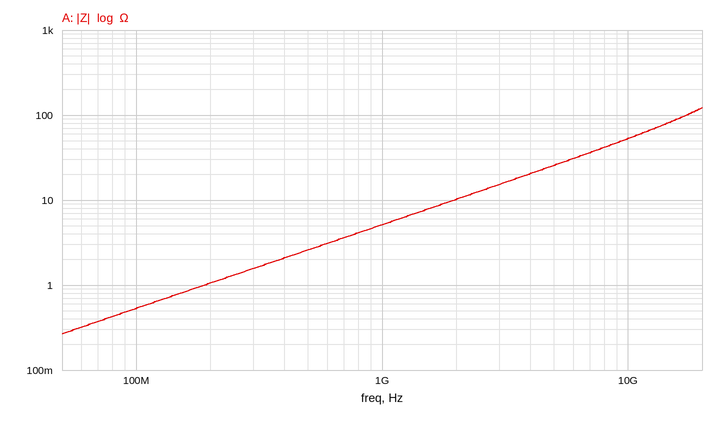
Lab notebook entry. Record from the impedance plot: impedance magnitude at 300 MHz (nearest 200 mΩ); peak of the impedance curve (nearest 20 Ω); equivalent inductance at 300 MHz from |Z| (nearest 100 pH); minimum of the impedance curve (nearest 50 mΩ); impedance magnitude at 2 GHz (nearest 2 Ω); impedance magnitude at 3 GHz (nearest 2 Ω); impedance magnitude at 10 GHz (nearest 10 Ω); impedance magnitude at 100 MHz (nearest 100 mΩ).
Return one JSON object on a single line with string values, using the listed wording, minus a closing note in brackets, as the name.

{"impedance magnitude at 300 MHz": "1.6 Ω", "peak of the impedance curve": "120 Ω", "equivalent inductance at 300 MHz from |Z|": "800 pH", "minimum of the impedance curve": "250 mΩ", "impedance magnitude at 2 GHz": "10 Ω", "impedance magnitude at 3 GHz": "16 Ω", "impedance magnitude at 10 GHz": "50 Ω", "impedance magnitude at 100 MHz": "500 mΩ"}
